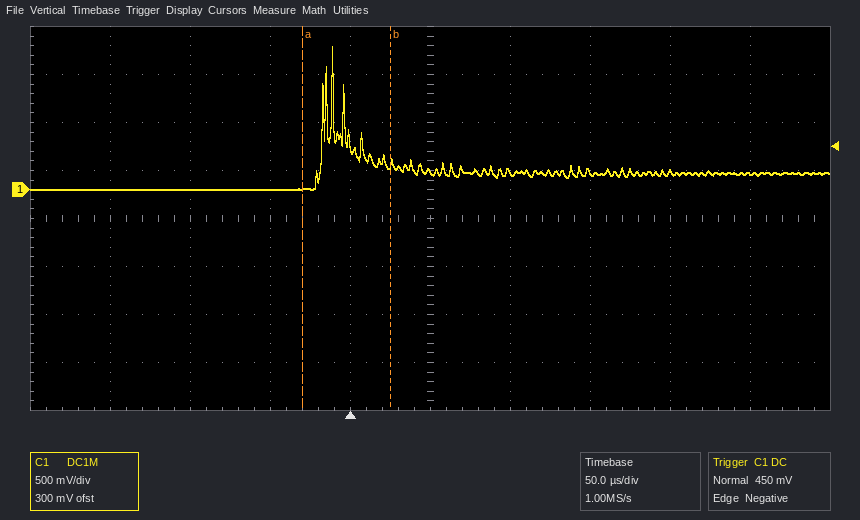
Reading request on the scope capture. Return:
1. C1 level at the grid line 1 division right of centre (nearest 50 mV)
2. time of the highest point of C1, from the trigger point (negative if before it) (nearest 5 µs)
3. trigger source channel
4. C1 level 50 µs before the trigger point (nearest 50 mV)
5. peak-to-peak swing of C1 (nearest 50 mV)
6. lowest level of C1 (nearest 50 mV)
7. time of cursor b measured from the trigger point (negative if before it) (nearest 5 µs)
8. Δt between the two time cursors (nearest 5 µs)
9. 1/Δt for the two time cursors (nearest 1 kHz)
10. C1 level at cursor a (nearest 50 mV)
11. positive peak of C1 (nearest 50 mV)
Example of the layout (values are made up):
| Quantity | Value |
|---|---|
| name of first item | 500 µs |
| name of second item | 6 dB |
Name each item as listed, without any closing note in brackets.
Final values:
| Quantity | Value |
|---|---|
| C1 level at the grid line 1 division right of centre | 200 mV |
| time of the highest point of C1, from the trigger point (negative if before it) | -10 µs |
| trigger source channel | C1 |
| C1 level 50 µs before the trigger point | 0 mV |
| peak-to-peak swing of C1 | 1.50 V |
| lowest level of C1 | 0 mV |
| time of cursor b measured from the trigger point (negative if before it) | +25 µs |
| Δt between the two time cursors | 55 µs |
| 1/Δt for the two time cursors | 18 kHz |
| C1 level at cursor a | 0 mV |
| positive peak of C1 | 1.50 V |
